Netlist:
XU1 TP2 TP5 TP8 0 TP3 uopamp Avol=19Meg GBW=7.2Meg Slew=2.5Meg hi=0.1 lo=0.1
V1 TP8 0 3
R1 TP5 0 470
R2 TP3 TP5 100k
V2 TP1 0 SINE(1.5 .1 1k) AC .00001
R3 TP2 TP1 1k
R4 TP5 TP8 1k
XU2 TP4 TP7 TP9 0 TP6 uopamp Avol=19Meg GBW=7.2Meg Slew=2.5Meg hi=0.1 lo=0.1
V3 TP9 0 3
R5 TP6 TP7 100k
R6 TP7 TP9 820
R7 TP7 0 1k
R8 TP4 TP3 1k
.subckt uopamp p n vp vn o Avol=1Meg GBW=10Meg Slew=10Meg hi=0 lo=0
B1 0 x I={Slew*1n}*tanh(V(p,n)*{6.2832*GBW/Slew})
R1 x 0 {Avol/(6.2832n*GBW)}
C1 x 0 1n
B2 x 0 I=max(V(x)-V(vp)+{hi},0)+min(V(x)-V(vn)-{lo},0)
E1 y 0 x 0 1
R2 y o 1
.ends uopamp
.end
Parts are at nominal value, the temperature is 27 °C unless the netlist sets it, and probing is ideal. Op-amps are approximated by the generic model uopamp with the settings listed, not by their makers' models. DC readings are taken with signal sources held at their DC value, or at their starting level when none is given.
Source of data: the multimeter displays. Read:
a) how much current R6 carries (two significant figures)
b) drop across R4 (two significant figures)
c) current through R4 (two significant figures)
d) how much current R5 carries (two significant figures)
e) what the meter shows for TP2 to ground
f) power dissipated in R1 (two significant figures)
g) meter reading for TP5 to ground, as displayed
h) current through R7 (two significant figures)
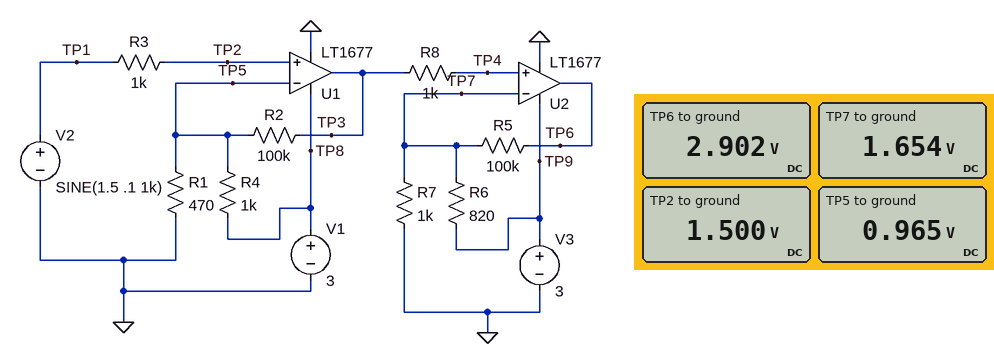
1.6 mA
2.0 V
2.0 mA
12 µA
1.500 V
2.0 mW
0.965 V
1.7 mA
